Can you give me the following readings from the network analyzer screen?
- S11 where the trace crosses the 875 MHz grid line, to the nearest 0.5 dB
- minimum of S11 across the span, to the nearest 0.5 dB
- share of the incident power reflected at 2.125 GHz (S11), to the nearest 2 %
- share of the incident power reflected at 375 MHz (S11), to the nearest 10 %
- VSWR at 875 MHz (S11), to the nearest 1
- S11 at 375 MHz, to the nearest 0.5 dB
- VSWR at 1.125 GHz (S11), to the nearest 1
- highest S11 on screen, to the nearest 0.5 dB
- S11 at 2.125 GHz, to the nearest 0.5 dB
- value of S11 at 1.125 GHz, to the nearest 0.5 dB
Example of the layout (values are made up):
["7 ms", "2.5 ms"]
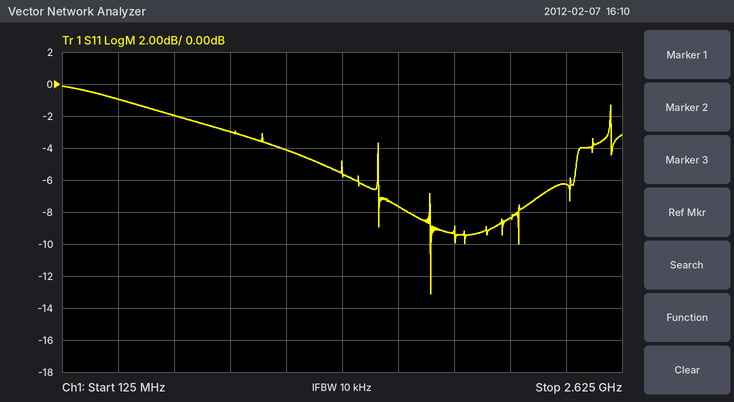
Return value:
["-3.0 dB", "-13.0 dB", "14 %", "80 %", "6", "-1.0 dB", "4", "0.0 dB", "-8.5 dB", "-4.0 dB"]
